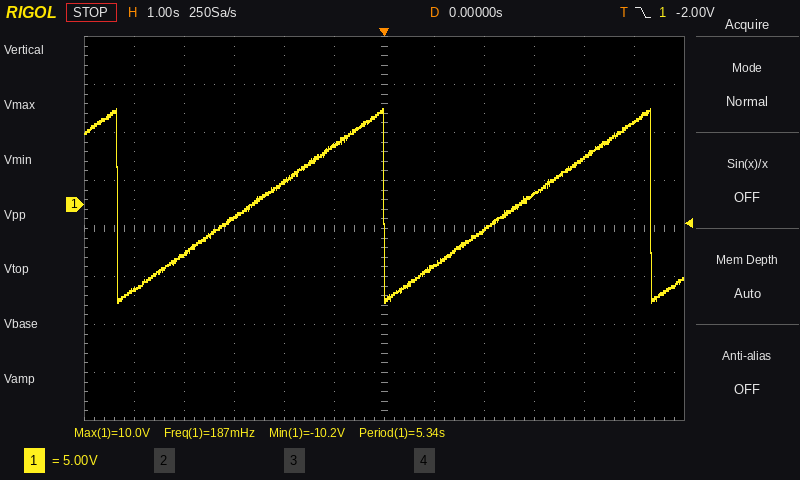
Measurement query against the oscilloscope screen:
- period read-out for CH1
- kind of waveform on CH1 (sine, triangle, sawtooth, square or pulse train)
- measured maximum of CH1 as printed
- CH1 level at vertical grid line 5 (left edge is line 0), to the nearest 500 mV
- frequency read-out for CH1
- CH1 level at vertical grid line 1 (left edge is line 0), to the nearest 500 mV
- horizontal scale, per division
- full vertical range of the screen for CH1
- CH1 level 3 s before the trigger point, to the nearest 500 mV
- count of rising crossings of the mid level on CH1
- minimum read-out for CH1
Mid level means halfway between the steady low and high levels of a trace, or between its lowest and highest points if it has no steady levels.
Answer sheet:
5.34 s
sawtooth
10.0 V
6.0 V
187 mHz
-9.0 V
1 s
40 V
-1.5 V
2
-10.2 V
